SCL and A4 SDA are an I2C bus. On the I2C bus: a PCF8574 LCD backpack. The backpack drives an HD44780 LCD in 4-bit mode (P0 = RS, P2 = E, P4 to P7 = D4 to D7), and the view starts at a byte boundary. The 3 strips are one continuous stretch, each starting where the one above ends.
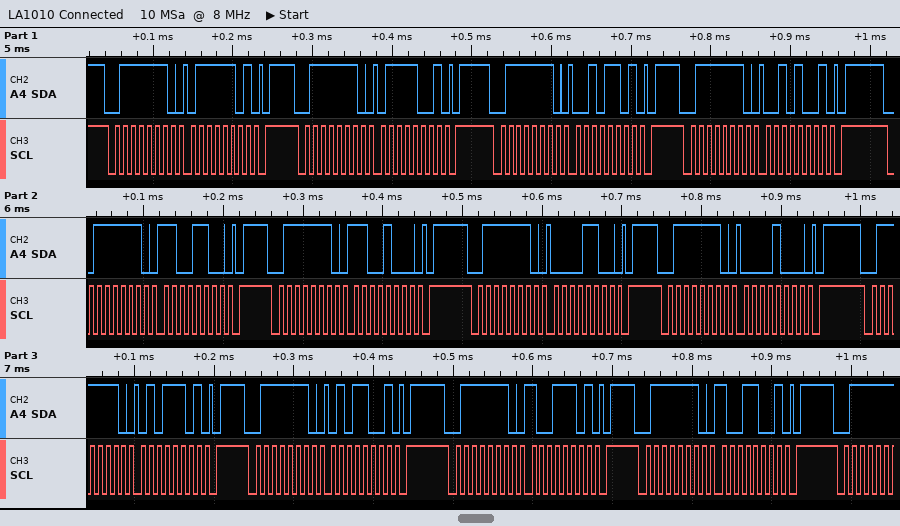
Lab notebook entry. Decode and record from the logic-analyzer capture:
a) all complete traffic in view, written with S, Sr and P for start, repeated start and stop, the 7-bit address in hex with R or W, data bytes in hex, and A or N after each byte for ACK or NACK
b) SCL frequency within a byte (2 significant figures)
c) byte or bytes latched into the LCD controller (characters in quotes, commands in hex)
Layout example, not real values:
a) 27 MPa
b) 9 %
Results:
a) S 3FW A 7D A P S 3FW A 79 A P S 3FW A 2D A P S 3FW A 29 A P S 3FW A CC A P S 3FW A C8 A P S 3FW A 0C A P S 3FW A 08 A P S 3FW A 5D A P S 3FW A 59 A P S 3FW A 9D A P S 3FW A 99 A P
b) 100 kHz
c) 'r' 0xC0 'Y'
